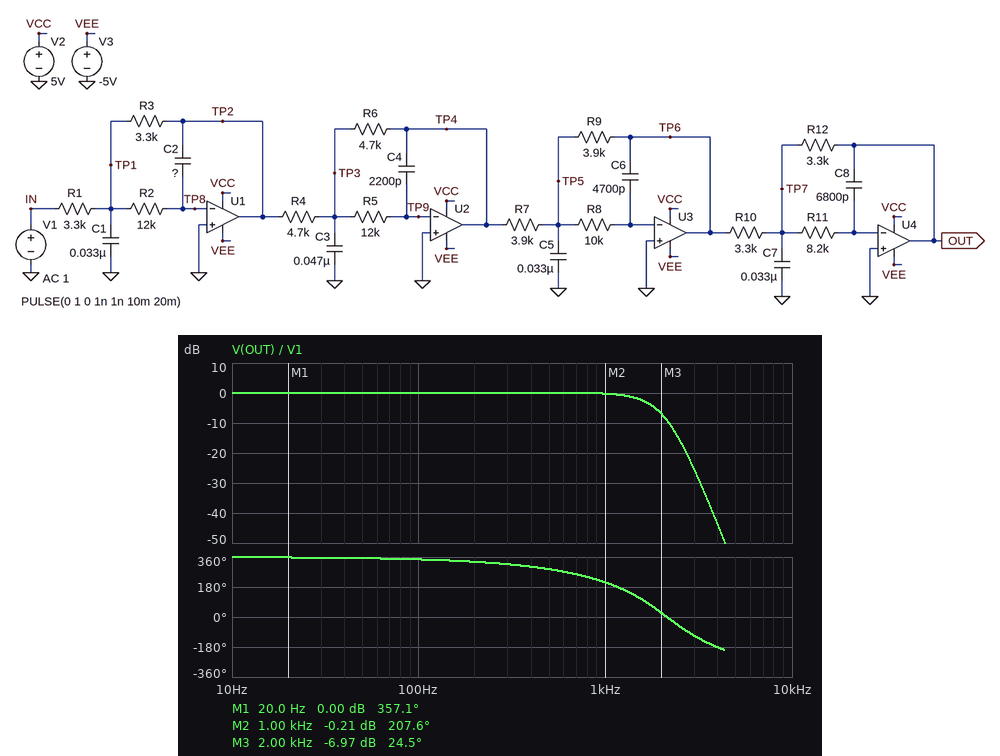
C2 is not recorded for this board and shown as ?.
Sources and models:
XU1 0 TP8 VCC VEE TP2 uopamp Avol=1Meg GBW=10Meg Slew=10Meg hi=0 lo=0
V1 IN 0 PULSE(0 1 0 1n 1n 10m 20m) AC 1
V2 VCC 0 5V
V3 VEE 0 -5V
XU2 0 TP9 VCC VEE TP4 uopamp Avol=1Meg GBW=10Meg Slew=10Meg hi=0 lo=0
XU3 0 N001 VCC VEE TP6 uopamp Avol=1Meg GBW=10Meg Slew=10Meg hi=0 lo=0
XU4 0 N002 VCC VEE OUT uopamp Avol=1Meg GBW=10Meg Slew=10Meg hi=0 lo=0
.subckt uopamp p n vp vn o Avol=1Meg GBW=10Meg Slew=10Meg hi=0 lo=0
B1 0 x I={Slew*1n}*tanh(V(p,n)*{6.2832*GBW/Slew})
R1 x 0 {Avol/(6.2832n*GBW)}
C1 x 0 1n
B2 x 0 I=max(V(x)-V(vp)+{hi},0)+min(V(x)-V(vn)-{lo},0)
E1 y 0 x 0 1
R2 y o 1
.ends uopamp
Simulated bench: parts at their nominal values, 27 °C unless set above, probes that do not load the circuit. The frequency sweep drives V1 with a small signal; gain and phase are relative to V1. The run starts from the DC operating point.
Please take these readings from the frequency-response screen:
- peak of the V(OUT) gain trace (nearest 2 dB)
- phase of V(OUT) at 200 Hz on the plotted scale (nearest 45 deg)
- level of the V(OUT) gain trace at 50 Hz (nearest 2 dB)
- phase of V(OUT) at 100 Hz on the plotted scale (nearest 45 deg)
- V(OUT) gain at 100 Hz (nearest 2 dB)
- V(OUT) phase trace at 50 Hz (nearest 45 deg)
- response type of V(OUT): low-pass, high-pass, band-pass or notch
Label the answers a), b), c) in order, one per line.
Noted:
a) 0 dB
b) 315 deg
c) 0 dB
d) 360 deg
e) 0 dB
f) 360 deg
g) low-pass
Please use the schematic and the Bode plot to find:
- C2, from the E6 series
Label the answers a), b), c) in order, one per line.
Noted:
a) 3.3 nF
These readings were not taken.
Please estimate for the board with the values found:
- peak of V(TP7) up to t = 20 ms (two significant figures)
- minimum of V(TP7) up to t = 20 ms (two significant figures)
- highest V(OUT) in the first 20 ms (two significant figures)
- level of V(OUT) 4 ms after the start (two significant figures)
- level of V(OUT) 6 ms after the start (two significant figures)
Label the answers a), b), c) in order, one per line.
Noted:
a) 220 mV
b) -220 mV
c) 1.1 V
d) 1.0 V
e) 1.0 V
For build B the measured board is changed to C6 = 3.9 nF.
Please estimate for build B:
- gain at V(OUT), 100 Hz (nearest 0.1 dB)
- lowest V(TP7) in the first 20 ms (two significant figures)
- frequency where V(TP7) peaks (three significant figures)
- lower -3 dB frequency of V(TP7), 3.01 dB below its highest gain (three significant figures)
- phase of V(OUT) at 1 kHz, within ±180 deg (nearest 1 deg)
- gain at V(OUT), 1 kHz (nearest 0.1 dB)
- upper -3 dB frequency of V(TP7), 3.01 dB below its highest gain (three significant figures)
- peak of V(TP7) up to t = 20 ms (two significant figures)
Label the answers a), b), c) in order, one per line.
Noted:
a) 0 dB
b) -230 mV
c) 1.55 kHz
d) 925 Hz
e) -146 deg
f) 0.2 dB
g) 2.10 kHz
h) 230 mV
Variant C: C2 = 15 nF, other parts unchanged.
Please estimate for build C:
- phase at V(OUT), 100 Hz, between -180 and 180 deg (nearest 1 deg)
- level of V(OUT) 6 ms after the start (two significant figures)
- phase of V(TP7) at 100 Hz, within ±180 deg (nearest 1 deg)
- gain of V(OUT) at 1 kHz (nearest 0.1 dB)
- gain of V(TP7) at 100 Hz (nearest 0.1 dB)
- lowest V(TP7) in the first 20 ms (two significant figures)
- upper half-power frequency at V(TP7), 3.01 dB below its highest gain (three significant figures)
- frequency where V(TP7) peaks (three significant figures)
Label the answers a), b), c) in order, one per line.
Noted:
a) -26 deg
b) 1.0 V
c) -116 deg
d) -8.4 dB
e) -29.3 dB
f) -100 mV
g) 1.72 kHz
h) 934 Hz
